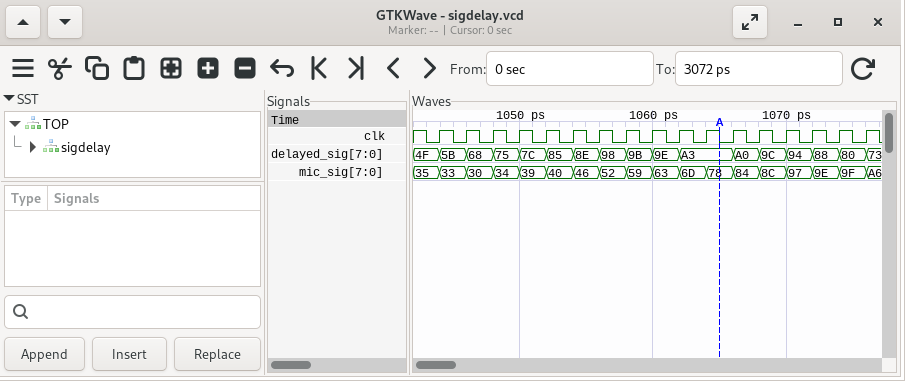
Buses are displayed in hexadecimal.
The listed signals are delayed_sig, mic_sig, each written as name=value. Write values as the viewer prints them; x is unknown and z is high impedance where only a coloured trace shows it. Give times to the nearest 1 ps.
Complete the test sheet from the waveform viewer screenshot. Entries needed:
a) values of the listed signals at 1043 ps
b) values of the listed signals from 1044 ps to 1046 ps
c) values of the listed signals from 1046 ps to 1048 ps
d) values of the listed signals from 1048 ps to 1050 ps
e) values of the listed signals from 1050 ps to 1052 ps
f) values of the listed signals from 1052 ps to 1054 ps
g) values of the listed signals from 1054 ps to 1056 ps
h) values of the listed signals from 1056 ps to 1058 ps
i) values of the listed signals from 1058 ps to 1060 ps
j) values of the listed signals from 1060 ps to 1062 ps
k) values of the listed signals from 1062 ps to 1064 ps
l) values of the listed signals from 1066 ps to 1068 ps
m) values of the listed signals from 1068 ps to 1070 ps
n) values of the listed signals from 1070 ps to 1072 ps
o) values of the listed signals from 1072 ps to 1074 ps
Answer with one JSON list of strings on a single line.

["delayed_sig=4F, mic_sig=35", "delayed_sig=5B, mic_sig=33", "delayed_sig=68, mic_sig=30", "delayed_sig=75, mic_sig=34", "delayed_sig=7C, mic_sig=39", "delayed_sig=85, mic_sig=40", "delayed_sig=8E, mic_sig=46", "delayed_sig=98, mic_sig=52", "delayed_sig=9B, mic_sig=59", "delayed_sig=9E, mic_sig=63", "delayed_sig=A3, mic_sig=6D", "delayed_sig=A0, mic_sig=84", "delayed_sig=9C, mic_sig=8C", "delayed_sig=94, mic_sig=97", "delayed_sig=88, mic_sig=9E"]
